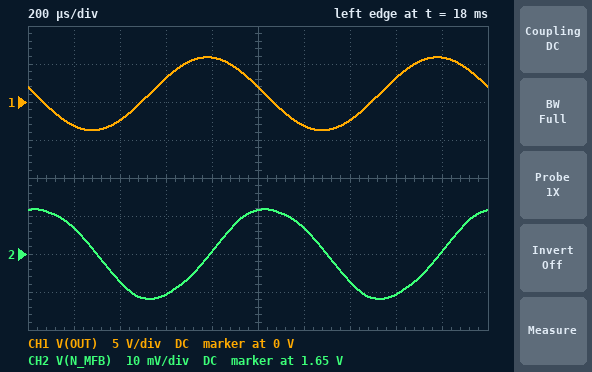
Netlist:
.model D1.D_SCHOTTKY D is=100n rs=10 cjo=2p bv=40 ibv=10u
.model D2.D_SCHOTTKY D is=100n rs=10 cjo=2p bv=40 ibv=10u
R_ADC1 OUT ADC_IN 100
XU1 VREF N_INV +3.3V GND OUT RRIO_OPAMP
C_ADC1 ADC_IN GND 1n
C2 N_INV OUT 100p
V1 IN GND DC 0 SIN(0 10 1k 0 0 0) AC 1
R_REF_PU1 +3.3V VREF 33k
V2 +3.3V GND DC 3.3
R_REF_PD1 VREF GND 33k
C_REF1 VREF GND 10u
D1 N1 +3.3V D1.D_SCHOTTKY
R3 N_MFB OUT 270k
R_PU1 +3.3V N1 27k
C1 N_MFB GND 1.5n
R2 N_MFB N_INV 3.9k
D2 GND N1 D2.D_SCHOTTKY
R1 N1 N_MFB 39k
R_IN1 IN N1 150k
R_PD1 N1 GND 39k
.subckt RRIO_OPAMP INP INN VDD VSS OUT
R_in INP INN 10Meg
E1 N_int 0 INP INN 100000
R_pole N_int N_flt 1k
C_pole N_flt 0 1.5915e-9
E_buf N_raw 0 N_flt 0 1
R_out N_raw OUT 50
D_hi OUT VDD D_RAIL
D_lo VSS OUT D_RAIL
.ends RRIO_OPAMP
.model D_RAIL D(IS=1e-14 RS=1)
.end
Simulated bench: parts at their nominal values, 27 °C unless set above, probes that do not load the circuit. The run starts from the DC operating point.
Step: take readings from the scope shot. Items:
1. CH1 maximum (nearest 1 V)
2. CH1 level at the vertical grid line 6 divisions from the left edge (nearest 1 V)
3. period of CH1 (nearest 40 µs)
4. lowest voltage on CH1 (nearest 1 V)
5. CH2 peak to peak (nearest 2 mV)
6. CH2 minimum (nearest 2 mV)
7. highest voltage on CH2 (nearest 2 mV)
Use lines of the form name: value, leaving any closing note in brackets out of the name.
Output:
CH1 maximum: 6 V
CH1 level at the vertical grid line 6 divisions from the left edge: -3 V
period of CH1: 1.00 ms
lowest voltage on CH1: -4 V
CH2 peak to peak: 24 mV
CH2 minimum: 1.638 V
highest voltage on CH2: 1.662 V
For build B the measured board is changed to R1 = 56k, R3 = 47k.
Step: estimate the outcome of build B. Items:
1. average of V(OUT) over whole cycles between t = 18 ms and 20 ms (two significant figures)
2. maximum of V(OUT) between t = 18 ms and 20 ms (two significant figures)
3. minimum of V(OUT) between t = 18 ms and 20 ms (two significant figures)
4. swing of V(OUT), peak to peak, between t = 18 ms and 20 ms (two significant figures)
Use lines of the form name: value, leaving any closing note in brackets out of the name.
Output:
average of V(OUT) over whole cycles between t = 18 ms and 20 ms: 1.6 V
maximum of V(OUT) between t = 18 ms and 20 ms: 2.2 V
minimum of V(OUT) between t = 18 ms and 20 ms: 930 mV
swing of V(OUT), peak to peak, between t = 18 ms and 20 ms: 1.3 V
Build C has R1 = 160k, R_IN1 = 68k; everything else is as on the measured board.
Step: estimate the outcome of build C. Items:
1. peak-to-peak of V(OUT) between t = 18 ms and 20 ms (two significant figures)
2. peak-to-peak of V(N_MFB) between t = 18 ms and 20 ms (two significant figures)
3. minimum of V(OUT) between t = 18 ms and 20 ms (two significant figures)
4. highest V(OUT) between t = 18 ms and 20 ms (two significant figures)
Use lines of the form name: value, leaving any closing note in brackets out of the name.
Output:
peak-to-peak of V(OUT) between t = 18 ms and 20 ms: 5.8 V
peak-to-peak of V(N_MFB) between t = 18 ms and 20 ms: 14 mV
minimum of V(OUT) between t = 18 ms and 20 ms: -1.2 V
highest V(OUT) between t = 18 ms and 20 ms: 4.6 V
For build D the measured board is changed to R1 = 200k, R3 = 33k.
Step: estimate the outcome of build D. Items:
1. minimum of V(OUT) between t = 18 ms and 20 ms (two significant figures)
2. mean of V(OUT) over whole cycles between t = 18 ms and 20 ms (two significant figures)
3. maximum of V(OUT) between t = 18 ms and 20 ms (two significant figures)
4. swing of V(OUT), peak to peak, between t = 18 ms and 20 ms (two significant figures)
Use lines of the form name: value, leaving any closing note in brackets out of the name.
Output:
minimum of V(OUT) between t = 18 ms and 20 ms: 1.5 V
mean of V(OUT) over whole cycles between t = 18 ms and 20 ms: 1.6 V
maximum of V(OUT) between t = 18 ms and 20 ms: 1.8 V
swing of V(OUT), peak to peak, between t = 18 ms and 20 ms: 300 mV
